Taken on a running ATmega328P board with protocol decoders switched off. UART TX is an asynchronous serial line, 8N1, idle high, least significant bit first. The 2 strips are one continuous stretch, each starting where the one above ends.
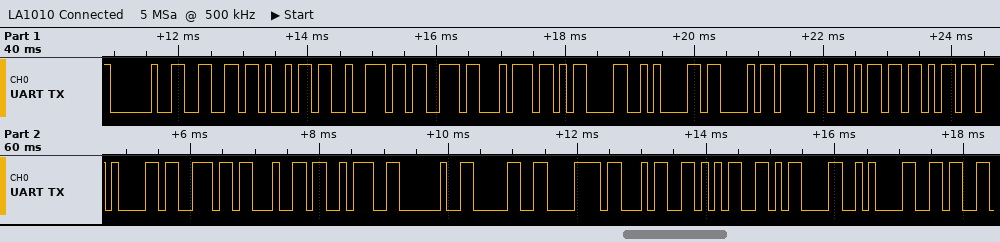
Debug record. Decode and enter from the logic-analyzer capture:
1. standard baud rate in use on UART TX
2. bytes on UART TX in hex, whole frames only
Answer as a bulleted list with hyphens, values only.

- 9600 baud
- 20 66 69 72 73 74 0D 0A 43 6F 6D 6D 61 6E 64 3A 20 30 78 34 35 0D 0A 36
